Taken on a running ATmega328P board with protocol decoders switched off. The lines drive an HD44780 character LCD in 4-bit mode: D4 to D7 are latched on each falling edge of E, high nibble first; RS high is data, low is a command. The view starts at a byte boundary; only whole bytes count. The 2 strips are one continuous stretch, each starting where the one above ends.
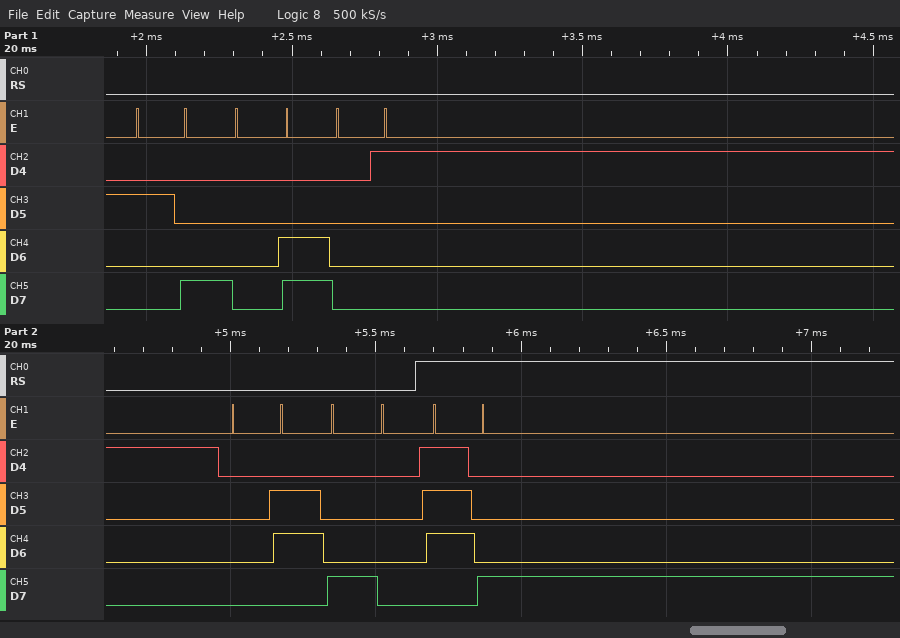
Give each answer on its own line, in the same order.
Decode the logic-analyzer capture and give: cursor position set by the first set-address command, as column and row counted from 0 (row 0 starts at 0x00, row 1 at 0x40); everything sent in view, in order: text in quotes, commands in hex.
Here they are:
column 0, row 0
0x28 0x0C 0x01 0x06 0x80 "x"
